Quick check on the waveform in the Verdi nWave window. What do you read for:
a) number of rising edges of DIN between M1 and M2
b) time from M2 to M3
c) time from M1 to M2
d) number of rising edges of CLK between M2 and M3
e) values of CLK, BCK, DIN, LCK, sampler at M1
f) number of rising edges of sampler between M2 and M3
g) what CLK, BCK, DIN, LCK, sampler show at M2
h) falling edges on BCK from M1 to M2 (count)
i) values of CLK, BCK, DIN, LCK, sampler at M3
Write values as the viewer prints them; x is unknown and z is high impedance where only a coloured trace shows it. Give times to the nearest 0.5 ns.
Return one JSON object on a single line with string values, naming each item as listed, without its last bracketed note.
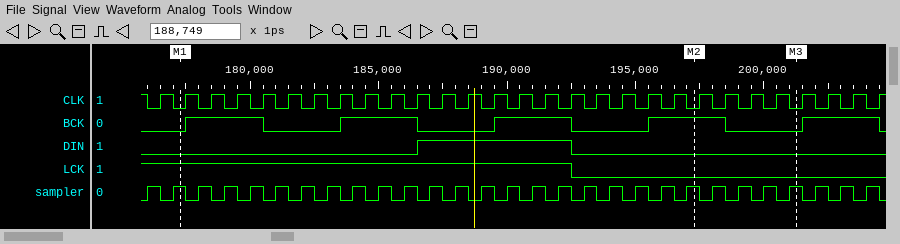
{"number of rising edges of DIN between M1 and M2": "1", "time from M2 to M3": "4 ns", "time from M1 to M2": "20 ns", "number of rising edges of CLK between M2 and M3": "4", "values of CLK, BCK, DIN, LCK, sampler at M1": "CLK=0, BCK=0, DIN=0, LCK=1, sampler=1", "number of rising edges of sampler between M2 and M3": "4", "what CLK, BCK, DIN, LCK, sampler show at M2": "CLK=0, BCK=1, DIN=0, LCK=0, sampler=1", "falling edges on BCK from M1 to M2": "3", "values of CLK, BCK, DIN, LCK, sampler at M3": "CLK=0, BCK=0, DIN=0, LCK=0, sampler=1"}
